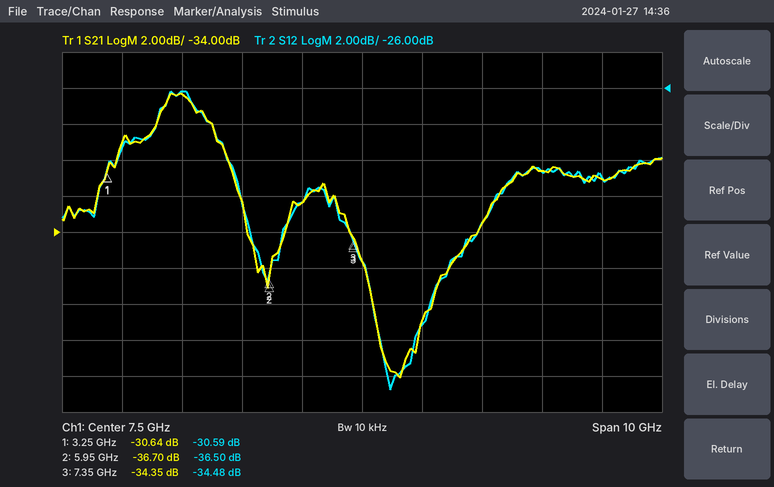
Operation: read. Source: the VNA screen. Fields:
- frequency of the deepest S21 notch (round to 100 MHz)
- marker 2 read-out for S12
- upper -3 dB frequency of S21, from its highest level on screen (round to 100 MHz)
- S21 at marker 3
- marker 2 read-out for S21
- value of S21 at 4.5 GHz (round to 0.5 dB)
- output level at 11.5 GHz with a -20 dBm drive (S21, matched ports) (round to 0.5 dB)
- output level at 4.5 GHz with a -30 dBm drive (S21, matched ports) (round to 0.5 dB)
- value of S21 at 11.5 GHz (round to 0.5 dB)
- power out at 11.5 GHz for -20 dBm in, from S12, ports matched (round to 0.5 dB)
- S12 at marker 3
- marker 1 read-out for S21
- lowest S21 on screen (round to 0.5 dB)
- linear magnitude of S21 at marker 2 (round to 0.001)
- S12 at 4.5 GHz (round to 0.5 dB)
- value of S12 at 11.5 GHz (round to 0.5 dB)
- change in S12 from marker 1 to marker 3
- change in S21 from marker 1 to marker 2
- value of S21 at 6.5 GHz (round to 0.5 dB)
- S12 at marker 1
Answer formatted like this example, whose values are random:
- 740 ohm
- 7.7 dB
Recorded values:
- 8.1 GHz
- -36.50 dB
- 5.2 GHz
- -34.35 dB
- -36.70 dB
- -26.5 dB
- -51.0 dBm
- -56.5 dBm
- -31.0 dB
- -51.0 dBm
- -34.48 dB
- -30.64 dB
- -42.0 dB
- 0.015
- -26.0 dB
- -31.0 dB
- -3.89 dB
- -6.06 dB
- -32.5 dB
- -30.59 dB
